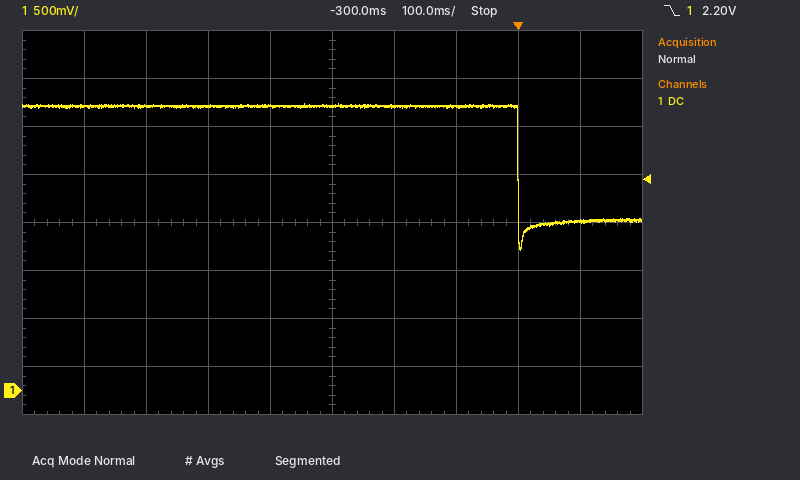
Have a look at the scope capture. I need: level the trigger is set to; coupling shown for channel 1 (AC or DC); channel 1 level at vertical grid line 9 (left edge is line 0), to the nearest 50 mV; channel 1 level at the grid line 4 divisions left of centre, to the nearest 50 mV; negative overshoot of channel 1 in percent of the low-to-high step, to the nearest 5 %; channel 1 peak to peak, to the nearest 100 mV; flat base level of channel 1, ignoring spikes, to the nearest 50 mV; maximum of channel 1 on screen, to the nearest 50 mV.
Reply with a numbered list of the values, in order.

1. 2.20 V
2. DC
3. 1.75 V
4. 2.95 V
5. 25 %
6. 1.50 V
7. 1.75 V
8. 3.00 V
